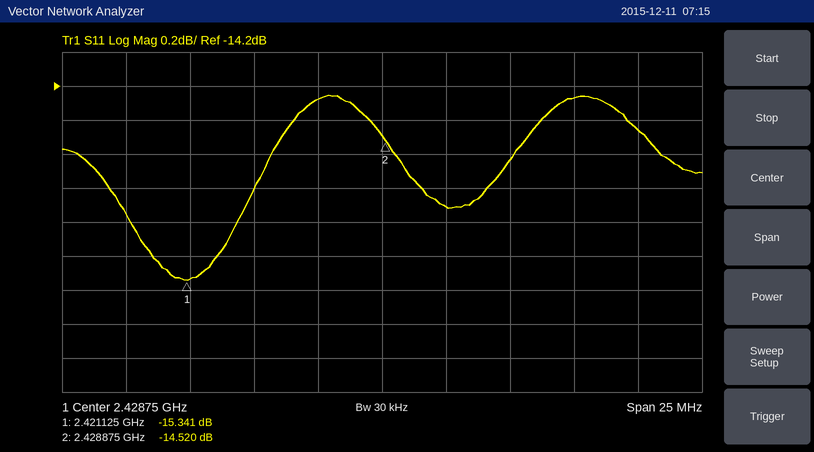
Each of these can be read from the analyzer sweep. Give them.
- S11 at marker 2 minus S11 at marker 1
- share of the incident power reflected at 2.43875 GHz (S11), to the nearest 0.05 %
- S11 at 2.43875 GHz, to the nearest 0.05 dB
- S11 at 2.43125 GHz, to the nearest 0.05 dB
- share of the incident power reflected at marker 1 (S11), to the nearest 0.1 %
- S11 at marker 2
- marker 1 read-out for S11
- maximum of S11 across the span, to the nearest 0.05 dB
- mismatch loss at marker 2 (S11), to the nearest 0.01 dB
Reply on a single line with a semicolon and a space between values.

0.821 dB; 3.60 %; -14.45 dB; -14.90 dB; 2.9 %; -14.520 dB; -15.341 dB; -14.25 dB; 0.16 dB
